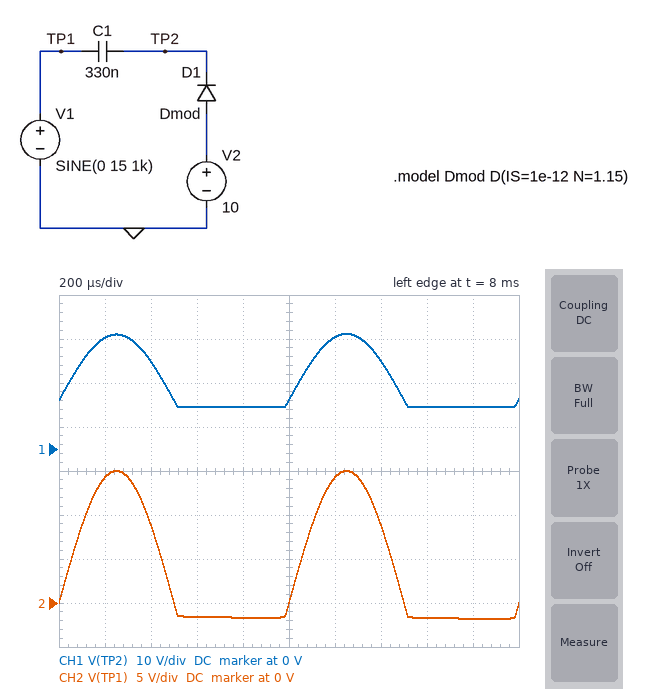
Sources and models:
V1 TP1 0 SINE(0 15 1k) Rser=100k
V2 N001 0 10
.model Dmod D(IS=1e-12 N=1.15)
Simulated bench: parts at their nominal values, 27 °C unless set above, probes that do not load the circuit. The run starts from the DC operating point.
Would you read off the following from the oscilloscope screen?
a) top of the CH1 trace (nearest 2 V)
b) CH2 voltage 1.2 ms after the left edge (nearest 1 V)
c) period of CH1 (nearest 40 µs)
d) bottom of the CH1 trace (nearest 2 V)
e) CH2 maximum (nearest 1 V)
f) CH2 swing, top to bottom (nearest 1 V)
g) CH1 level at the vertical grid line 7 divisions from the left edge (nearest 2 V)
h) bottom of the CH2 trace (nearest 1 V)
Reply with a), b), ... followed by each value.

a) 26 V
b) 14 V
c) 1.00 ms
d) 10 V
e) 15 V
f) 17 V
g) 20 V
h) -2 V
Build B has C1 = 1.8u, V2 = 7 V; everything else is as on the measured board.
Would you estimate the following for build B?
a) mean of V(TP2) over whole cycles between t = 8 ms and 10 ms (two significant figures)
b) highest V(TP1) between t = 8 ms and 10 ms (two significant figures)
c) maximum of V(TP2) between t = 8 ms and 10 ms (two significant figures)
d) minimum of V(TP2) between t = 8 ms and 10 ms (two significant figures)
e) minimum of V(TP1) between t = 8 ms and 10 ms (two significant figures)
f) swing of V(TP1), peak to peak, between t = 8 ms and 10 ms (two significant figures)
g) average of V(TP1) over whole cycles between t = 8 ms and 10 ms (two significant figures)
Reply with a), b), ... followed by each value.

a) 12 V
b) 15 V
c) 22 V
d) 6.4 V
e) -800 mV
f) 16 V
g) 4.4 V
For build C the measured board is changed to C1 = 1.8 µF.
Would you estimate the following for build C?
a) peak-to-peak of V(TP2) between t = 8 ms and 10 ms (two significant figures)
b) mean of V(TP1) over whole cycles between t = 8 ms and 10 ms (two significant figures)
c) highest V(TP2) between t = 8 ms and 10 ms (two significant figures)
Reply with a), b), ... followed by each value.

a) 16 V
b) 4.4 V
c) 25 V
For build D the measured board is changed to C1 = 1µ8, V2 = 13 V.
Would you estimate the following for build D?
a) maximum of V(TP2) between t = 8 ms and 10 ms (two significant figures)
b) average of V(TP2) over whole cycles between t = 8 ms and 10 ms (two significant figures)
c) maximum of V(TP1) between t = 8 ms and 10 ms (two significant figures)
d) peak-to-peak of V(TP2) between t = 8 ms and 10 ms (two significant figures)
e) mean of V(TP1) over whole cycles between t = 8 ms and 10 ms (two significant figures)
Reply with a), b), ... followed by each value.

a) 28 V
b) 18 V
c) 15 V
d) 16 V
e) 4.4 V
